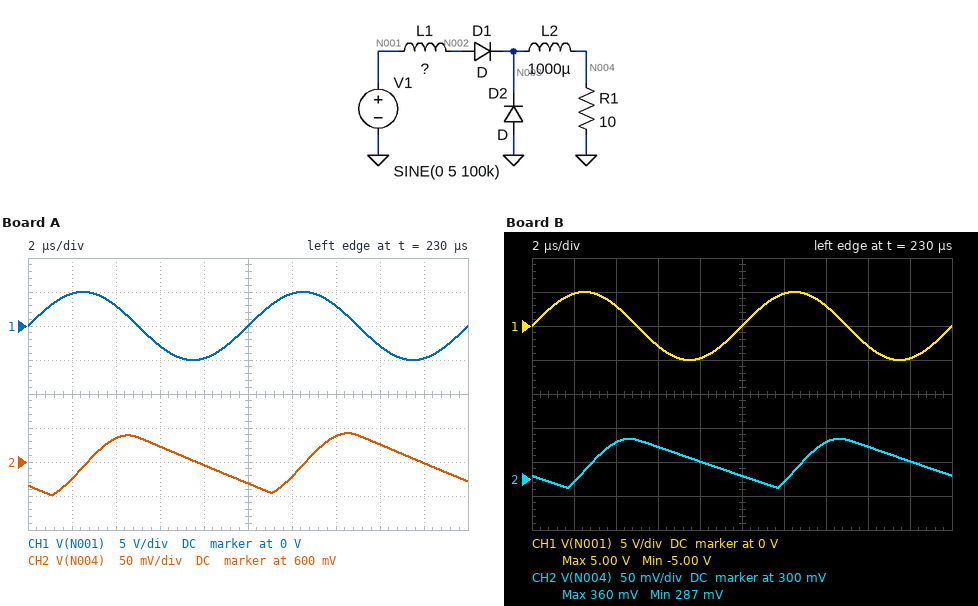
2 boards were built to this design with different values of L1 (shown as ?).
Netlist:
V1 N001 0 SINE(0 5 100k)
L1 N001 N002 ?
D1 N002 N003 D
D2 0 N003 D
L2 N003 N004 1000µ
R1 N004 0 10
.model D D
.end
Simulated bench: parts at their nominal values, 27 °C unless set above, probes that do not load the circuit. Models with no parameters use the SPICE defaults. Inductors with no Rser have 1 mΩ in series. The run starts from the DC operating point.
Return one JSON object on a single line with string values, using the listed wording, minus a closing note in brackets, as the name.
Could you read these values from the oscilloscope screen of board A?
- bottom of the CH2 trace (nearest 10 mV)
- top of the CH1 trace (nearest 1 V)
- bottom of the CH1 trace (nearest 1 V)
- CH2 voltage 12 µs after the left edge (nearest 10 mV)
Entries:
{"bottom of the CH2 trace": "550 mV", "top of the CH1 trace": "5 V", "bottom of the CH1 trace": "-5 V", "CH2 voltage 12 µs after the left edge": "580 mV"}
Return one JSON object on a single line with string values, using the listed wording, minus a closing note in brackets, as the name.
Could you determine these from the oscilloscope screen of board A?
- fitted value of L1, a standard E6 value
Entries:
{"fitted value of L1, a standard E6 value": "33 µH"}
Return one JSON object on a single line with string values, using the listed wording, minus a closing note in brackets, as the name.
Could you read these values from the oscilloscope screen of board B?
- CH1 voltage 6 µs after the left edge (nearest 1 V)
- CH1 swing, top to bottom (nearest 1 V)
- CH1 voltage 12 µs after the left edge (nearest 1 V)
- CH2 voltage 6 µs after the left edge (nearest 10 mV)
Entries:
{"CH1 voltage 6 µs after the left edge": "-3 V", "CH1 swing, top to bottom": "10 V", "CH1 voltage 12 µs after the left edge": "5 V", "CH2 voltage 6 µs after the left edge": "350 mV"}
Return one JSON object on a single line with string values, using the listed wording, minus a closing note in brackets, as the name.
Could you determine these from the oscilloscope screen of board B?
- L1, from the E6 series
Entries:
{"L1, from the E6 series": "150 µH"}
